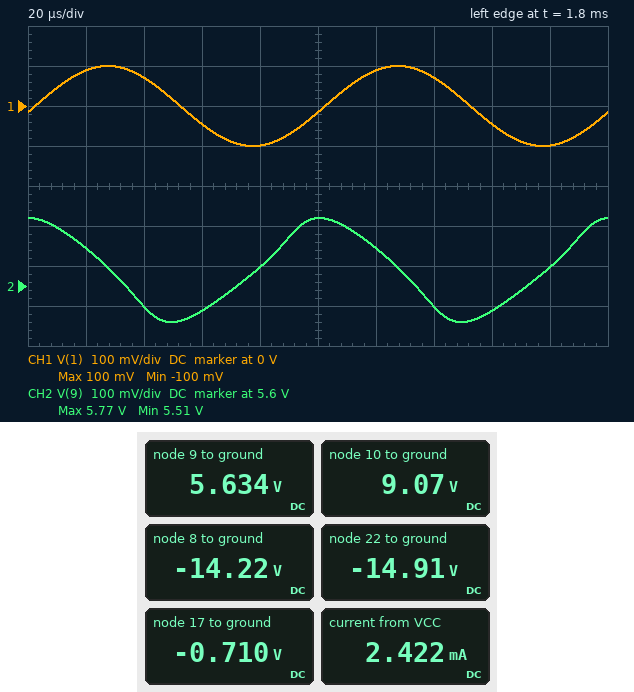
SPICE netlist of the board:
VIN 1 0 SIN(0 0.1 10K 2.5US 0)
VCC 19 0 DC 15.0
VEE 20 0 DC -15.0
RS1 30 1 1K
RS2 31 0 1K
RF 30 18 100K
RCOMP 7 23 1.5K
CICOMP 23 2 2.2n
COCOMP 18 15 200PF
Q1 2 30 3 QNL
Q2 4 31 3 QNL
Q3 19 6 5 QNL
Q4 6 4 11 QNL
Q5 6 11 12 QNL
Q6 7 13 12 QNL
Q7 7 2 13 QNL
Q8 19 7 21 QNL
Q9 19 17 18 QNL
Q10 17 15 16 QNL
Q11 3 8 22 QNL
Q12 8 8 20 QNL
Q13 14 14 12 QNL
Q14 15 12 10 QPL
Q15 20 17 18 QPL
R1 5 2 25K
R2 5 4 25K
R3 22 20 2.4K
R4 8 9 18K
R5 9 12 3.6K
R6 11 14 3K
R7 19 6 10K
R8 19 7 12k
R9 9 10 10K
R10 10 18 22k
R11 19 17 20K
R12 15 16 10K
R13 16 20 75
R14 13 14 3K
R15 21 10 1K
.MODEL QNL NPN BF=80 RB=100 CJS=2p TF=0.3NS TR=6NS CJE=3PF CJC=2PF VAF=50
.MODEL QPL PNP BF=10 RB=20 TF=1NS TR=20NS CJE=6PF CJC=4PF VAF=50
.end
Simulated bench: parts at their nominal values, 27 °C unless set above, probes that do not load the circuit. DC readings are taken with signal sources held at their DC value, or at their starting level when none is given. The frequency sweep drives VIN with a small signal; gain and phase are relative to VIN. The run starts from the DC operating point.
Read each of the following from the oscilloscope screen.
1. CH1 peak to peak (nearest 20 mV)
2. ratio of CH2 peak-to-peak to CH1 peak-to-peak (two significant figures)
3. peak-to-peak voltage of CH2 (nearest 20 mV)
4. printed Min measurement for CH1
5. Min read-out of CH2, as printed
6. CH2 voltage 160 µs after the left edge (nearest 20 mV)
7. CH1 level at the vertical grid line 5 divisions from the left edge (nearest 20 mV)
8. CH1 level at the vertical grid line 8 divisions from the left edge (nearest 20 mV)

200 mV
1.3
260 mV
-100 mV
5.51 V
5.54 V
-20 mV
-40 mV
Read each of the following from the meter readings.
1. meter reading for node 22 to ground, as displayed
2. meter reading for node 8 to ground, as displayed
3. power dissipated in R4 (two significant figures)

-14.91 V
-14.22 V
22 mW
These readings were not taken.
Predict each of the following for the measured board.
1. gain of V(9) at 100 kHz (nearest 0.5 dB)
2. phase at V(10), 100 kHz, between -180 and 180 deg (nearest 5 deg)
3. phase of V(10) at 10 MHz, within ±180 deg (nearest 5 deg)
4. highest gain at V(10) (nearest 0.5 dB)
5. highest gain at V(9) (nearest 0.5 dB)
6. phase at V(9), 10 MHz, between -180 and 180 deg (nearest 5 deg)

-1.0 dB
10 deg
-125 deg
6.0 dB
4.5 dB
-135 deg
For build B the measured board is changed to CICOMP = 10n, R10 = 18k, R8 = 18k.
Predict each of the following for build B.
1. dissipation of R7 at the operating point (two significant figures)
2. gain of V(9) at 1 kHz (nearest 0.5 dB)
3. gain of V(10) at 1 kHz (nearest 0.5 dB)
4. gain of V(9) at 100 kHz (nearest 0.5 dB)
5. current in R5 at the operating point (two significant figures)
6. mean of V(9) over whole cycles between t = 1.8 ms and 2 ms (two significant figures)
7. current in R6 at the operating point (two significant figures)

2.2 mW
3.5 dB
5.0 dB
0.5 dB
740 µA
5.1 V
21 µA
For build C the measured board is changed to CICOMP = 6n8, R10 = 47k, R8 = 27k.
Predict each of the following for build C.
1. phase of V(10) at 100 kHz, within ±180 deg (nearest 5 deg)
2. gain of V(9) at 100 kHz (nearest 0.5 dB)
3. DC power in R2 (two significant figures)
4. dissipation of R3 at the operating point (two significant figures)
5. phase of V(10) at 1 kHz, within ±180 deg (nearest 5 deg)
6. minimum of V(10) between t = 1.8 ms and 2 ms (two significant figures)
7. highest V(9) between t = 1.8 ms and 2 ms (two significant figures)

5 deg
2.5 dB
8.5 µW
3.6 µW
150 deg
7.9 V
4.8 V
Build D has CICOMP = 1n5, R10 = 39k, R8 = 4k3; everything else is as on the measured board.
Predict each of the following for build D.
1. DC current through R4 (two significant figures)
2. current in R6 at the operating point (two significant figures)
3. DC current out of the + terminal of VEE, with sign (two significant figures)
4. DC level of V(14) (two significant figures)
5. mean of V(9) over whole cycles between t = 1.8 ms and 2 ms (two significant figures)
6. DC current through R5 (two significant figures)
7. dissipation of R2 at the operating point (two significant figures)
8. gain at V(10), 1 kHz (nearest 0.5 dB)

1.2 mA
14 µA
-2.4 mA
11 V
7.3 V
820 µA
11 µW
5.0 dB
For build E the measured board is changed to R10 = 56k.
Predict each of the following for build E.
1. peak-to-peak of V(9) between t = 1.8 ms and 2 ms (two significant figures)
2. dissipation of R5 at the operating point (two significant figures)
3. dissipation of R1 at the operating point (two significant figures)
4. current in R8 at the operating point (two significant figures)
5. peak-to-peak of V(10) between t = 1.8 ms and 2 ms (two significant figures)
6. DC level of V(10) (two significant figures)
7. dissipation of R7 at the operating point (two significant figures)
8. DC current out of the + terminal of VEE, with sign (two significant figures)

240 mV
2.1 mW
9.5 µW
370 µA
350 mV
9.2 V
1.5 mW
-2.2 mA
